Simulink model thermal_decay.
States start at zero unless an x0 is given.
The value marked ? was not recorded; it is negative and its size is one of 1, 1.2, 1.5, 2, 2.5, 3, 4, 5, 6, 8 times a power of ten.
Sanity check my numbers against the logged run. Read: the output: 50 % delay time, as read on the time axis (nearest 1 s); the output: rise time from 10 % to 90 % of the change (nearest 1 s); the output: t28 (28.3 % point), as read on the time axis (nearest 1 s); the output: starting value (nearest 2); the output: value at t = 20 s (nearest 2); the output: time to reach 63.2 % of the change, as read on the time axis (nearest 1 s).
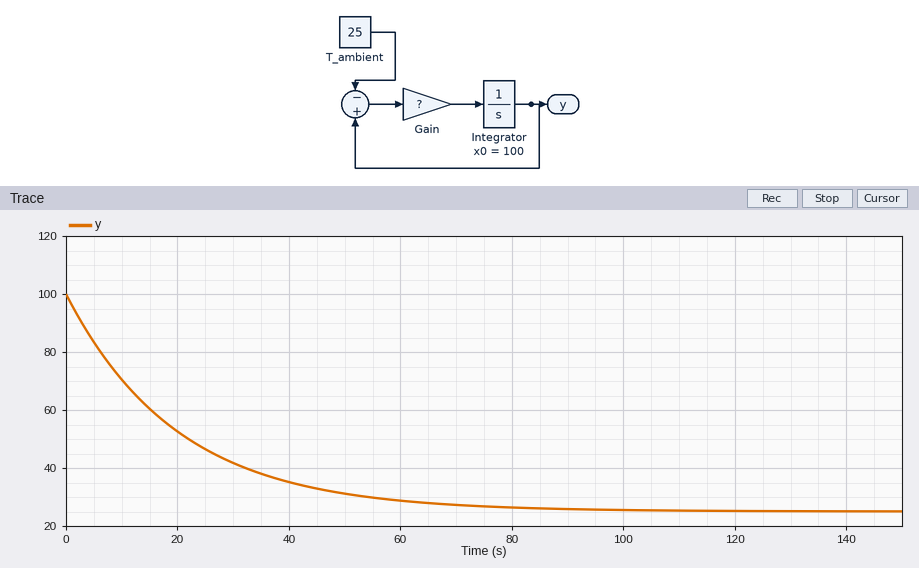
14 s
44 s
7 s
100
52
20 s
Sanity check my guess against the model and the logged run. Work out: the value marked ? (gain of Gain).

-0.05
